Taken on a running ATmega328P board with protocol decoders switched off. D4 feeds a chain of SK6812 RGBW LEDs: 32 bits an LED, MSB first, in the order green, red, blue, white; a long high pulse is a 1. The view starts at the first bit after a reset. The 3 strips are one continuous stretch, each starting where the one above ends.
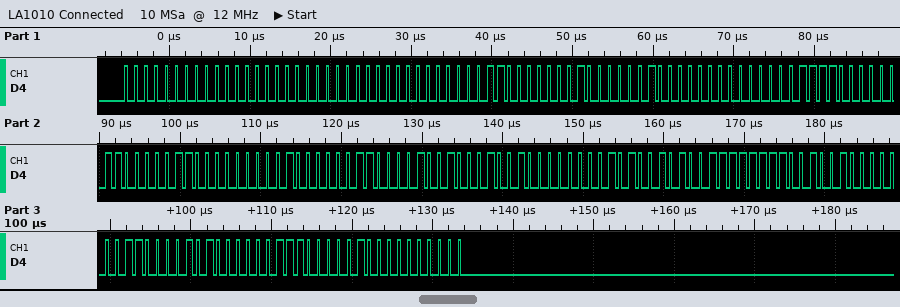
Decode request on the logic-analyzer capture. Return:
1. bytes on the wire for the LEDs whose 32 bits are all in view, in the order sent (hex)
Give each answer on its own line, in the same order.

00 00 00 00 0C 04 08 00 1E 06 0C 01 03 09 12 01 4A 7F 92 03 0A 07 04 00
